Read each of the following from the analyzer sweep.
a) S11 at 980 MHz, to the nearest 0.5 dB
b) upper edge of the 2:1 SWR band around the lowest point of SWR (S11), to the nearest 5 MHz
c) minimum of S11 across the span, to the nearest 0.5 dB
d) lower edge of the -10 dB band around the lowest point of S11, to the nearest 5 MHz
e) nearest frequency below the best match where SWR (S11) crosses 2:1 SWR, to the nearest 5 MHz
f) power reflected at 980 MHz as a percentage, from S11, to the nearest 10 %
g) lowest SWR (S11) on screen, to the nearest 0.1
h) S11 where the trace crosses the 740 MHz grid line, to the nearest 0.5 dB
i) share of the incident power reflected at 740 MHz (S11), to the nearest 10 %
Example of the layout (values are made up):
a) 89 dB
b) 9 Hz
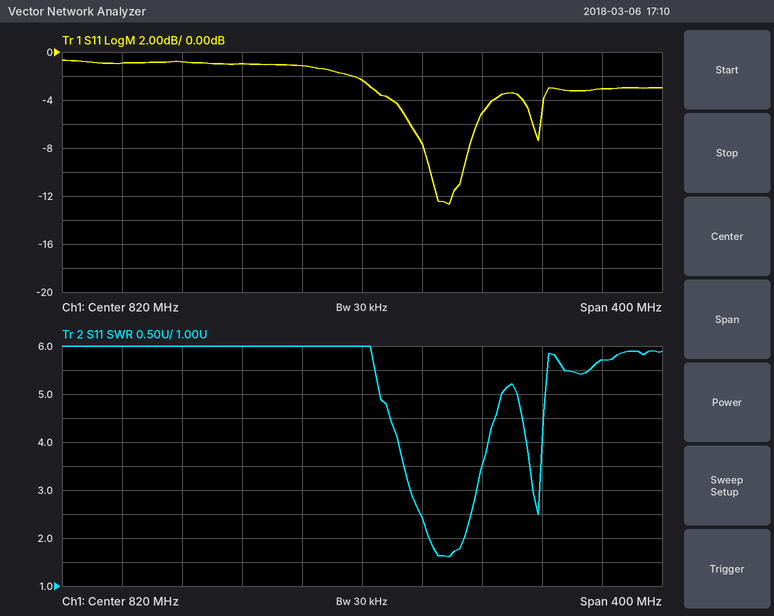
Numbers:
a) -3.0 dB
b) 890 MHz
c) -12.5 dB
d) 865 MHz
e) 865 MHz
f) 50 %
g) 1.6
h) -1.0 dB
i) 80 %
